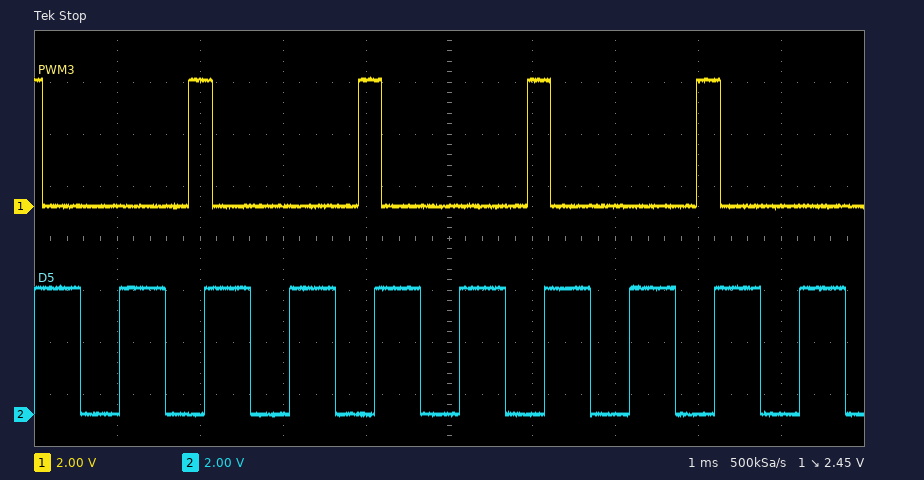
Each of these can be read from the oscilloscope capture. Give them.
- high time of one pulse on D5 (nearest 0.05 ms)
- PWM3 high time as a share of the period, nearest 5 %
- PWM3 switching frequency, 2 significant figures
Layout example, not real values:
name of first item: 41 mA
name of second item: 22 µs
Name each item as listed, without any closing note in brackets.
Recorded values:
high time of one pulse on D5: 0.55 ms
PWM3 high time as a share of the period, nearest 5 %: 15 %
PWM3 switching frequency, 2 significant figures: 490 Hz
